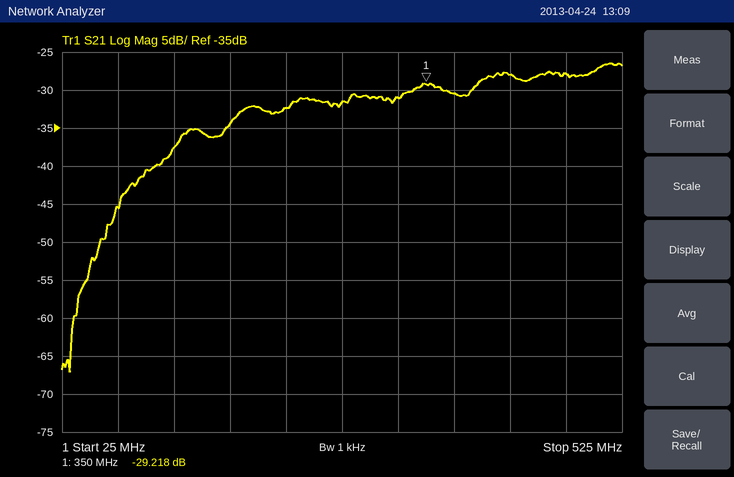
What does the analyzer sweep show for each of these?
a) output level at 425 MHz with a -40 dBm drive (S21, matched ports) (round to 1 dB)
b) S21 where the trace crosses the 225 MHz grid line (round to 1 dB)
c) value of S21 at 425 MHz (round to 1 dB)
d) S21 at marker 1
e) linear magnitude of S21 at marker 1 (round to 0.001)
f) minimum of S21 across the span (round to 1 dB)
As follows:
-68 dBm
-32 dB
-28 dB
-29.218 dB
0.035
-67 dB
